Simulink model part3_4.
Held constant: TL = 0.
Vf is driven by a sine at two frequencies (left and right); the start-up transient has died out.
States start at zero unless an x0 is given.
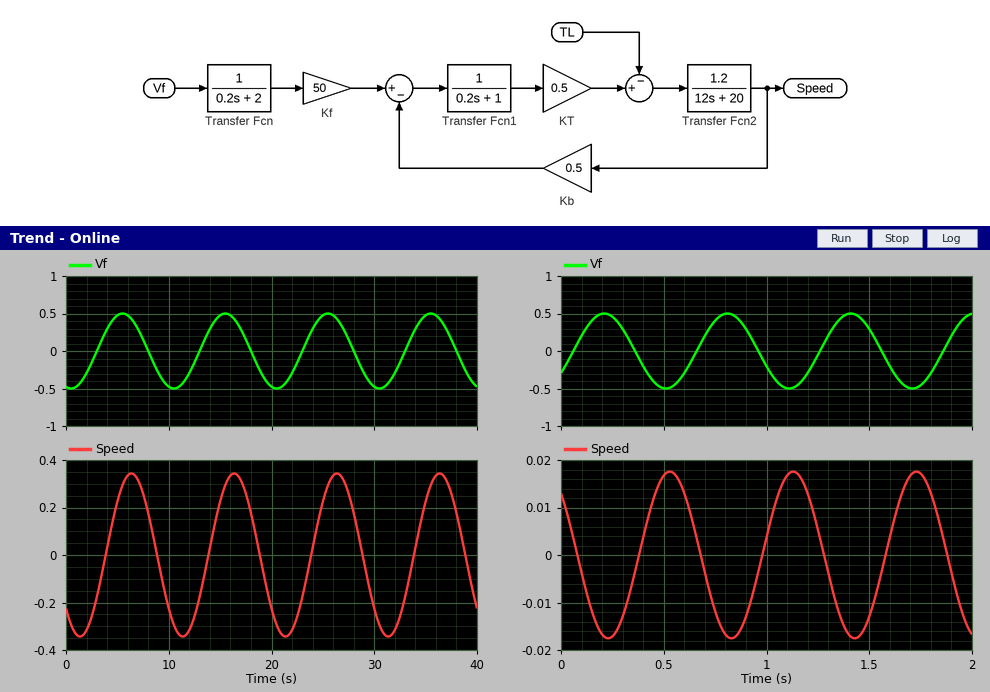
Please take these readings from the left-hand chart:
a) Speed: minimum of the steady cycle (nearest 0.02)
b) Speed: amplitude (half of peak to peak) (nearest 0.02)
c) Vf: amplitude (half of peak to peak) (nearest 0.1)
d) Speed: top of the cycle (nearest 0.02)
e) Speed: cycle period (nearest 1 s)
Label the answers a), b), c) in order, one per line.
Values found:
a) -0.34
b) 0.34
c) 0.5
d) 0.34
e) 10 s
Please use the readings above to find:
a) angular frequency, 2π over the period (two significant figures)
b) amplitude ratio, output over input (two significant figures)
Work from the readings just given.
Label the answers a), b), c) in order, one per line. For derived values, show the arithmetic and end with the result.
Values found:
a) 2π / 10 = 0.63 rad/s
b) 0.34 / 0.5 = 0.68
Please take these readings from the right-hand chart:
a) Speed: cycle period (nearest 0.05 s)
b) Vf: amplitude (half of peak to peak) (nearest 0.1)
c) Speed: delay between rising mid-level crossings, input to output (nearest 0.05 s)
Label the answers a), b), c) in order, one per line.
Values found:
a) 0.60 s
b) 0.5
c) 0.30 s
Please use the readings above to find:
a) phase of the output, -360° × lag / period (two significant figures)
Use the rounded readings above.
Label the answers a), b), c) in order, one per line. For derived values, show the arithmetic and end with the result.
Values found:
a) -360 × 0.3 / 0.6 = -180°
